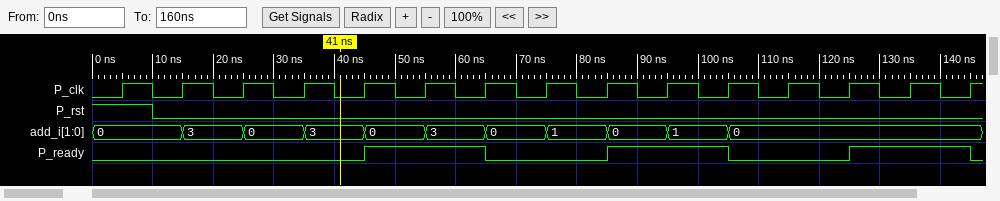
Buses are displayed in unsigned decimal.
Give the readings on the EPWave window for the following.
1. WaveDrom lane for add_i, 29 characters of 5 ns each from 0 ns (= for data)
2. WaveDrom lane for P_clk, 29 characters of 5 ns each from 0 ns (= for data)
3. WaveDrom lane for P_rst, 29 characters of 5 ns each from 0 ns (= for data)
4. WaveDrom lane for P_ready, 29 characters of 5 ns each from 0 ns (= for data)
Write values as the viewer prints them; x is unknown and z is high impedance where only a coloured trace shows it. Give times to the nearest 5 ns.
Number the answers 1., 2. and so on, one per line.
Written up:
1. {name: 'add_i', wave: '=..=.=.=.=.=.=.=.=.=.=.......', data: '0 3 0 3 0 3 0 1 0 1 0'}
2. {name: 'P_clk', wave: '01010101010101010101010101010'}
3. {name: 'P_rst', wave: '1.0..........................'}
4. {name: 'P_ready', wave: '0........1...0...1...0...1...'}
